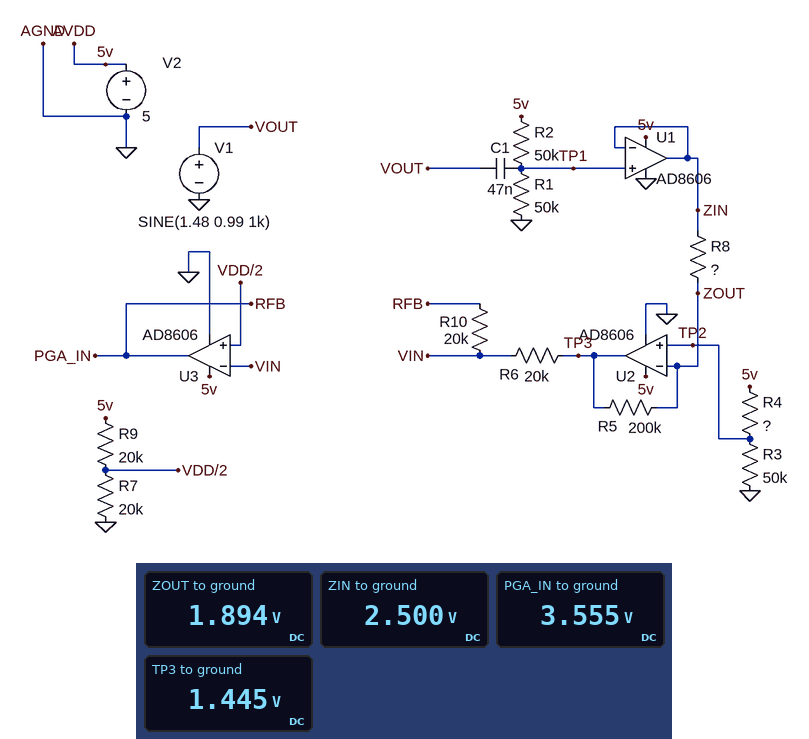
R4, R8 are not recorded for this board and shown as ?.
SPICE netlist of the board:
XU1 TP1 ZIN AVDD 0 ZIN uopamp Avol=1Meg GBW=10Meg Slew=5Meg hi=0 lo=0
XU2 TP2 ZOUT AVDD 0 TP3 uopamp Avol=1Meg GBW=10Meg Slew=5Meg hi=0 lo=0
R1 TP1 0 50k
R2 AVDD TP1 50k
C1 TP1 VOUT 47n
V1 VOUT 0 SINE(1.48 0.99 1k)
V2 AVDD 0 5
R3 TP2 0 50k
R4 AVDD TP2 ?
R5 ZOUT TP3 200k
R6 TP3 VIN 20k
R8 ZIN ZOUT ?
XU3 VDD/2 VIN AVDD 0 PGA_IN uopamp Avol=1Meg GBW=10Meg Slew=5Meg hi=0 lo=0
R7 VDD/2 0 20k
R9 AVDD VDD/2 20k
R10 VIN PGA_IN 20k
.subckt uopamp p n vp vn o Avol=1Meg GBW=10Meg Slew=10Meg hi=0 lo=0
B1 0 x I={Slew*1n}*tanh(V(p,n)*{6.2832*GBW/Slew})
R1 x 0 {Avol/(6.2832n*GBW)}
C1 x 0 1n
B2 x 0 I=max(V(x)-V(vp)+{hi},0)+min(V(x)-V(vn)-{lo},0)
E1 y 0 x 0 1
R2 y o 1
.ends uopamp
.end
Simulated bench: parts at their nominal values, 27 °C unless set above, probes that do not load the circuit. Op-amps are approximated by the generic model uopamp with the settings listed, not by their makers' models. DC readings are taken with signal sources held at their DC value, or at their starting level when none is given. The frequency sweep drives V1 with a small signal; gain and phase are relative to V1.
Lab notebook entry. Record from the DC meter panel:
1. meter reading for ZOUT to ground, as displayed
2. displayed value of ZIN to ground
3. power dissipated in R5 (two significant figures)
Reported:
1.894 V
2.500 V
1.0 µW
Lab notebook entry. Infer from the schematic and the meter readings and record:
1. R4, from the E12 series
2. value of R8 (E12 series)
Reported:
82 kΩ
270 kΩ
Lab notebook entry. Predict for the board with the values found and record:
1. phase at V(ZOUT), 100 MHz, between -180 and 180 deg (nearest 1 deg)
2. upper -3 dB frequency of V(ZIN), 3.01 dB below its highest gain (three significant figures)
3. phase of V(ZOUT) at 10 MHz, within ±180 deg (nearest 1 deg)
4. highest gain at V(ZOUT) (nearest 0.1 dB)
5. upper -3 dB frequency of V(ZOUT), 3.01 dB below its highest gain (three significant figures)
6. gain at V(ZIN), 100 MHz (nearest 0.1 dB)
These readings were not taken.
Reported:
-81 deg
10.0 MHz
-15 deg
-11.4 dB
18.8 MHz
-20.0 dB
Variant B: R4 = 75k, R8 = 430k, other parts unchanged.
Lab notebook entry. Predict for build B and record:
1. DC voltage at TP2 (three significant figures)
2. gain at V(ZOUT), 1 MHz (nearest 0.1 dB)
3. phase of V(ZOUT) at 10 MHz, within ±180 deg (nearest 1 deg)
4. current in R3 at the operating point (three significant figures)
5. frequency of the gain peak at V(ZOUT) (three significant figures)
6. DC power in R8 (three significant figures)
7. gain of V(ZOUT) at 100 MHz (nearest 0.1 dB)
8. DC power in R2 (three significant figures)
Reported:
2.00 V
-26.8 dB
-11 deg
40.0 µA
8.26 MHz
581 nW
-30.0 dB
125 µW
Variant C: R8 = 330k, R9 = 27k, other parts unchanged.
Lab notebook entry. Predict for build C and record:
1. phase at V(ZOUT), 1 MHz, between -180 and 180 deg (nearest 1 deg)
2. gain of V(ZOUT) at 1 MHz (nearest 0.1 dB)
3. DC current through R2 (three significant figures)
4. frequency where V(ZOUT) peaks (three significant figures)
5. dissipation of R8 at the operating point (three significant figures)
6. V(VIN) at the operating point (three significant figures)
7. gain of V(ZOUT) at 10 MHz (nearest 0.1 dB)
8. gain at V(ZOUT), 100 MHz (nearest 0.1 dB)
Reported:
75 deg
-24.5 dB
50.0 µA
7.89 MHz
1.11 µW
2.13 V
-12.9 dB
-28.5 dB
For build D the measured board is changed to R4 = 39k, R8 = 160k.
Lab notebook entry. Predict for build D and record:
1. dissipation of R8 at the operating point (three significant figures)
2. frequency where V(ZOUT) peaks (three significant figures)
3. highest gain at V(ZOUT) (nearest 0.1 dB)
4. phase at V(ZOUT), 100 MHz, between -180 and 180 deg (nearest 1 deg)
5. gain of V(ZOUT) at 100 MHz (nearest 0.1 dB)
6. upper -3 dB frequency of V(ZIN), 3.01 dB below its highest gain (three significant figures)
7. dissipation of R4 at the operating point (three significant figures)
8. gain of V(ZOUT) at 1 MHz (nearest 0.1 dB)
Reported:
597 nW
6.67 MHz
-8.3 dB
-82 deg
-25.2 dB
10.0 MHz
123 µW
-18.3 dB
